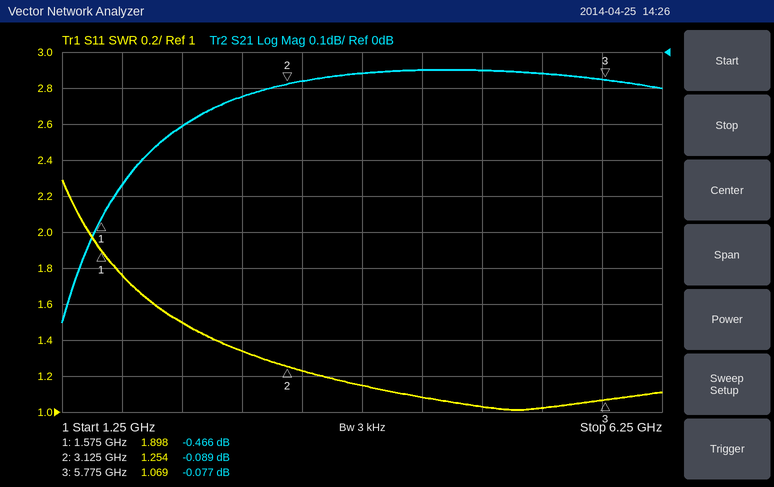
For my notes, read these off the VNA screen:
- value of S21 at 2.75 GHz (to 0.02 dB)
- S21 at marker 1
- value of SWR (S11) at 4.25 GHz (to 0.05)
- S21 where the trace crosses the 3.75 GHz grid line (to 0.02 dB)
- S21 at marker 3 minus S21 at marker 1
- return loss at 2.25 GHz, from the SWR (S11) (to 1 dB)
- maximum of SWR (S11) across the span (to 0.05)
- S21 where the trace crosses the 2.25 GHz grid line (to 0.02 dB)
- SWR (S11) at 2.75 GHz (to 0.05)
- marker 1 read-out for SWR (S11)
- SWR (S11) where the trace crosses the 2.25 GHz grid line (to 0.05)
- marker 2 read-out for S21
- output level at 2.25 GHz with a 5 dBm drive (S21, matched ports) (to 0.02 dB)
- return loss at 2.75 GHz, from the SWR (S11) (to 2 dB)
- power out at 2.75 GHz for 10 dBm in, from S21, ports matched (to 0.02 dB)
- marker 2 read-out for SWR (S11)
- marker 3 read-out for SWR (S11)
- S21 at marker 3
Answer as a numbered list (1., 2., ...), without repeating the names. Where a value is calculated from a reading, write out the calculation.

1. -0.12 dB
2. -0.466 dB
3. 1.10
4. -0.06 dB
5. -0.077 − (-0.466) = 0.389 dB
6. −20 log10((1.5 − 1)/(1.5 + 1)) ≈ 14 dB
7. 2.30
8. -0.20 dB
9. 1.35
10. 1.898
11. 1.50
12. -0.089 dB
13. 5 dBm + (-0.20 dB) = 4.80 dBm
14. −20 log10((1.35 − 1)/(1.35 + 1)) ≈ 16 dB
15. 10 dBm + (-0.12 dB) = 9.88 dBm
16. 1.254
17. 1.069
18. -0.077 dB
